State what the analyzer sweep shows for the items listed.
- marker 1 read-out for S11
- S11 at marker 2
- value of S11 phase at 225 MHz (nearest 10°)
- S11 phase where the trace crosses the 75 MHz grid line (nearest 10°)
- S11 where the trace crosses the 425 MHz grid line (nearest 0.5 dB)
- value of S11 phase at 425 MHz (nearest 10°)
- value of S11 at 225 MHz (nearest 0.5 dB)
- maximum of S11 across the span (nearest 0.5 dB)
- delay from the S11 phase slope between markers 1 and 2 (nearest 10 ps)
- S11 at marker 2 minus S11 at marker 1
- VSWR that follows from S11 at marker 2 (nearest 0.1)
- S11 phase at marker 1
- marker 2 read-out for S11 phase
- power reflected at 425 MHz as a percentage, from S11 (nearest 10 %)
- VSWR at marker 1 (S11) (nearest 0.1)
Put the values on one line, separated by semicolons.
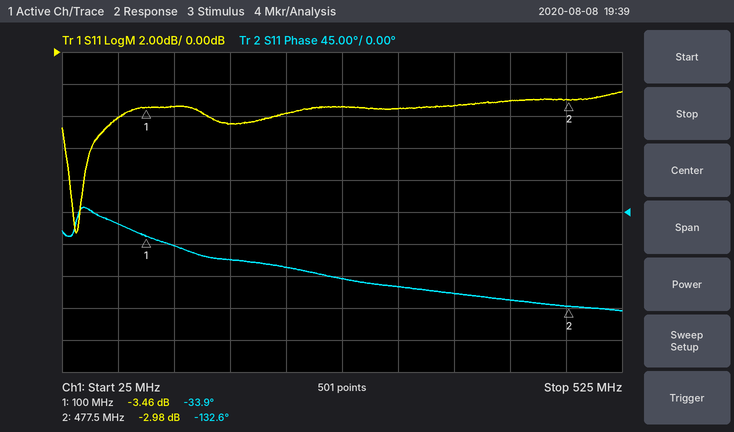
-3.46 dB; -2.98 dB; -80°; -20°; -3.0 dB; -120°; -4.0 dB; -2.5 dB; 730 ps; 0.48 dB; 5.9; -33.9°; -132.6°; 50 %; 5.1
